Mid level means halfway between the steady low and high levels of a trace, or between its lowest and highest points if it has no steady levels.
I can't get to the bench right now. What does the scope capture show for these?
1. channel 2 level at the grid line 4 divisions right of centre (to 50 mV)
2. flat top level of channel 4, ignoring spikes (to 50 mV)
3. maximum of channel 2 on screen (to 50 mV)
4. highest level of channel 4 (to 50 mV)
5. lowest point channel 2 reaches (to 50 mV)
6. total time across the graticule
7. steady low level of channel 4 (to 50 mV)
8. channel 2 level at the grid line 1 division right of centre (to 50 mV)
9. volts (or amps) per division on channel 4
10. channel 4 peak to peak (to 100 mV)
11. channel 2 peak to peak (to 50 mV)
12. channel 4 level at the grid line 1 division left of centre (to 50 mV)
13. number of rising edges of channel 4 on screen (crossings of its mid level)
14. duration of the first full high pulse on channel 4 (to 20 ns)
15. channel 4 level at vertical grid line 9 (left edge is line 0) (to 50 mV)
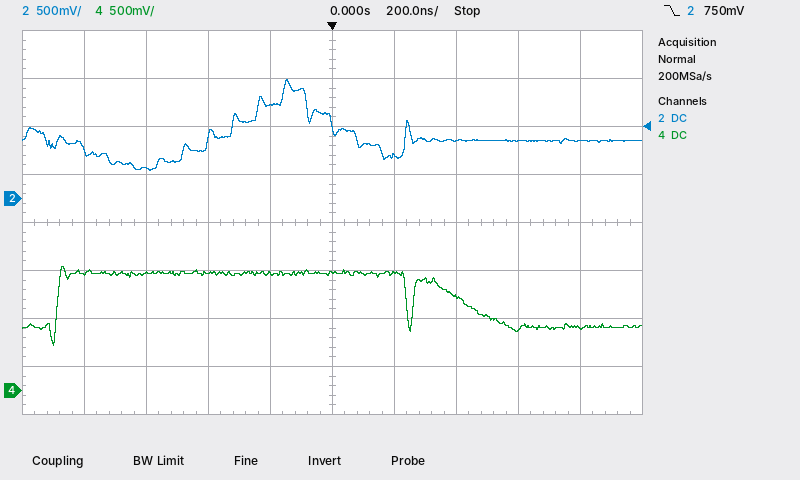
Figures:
600 mV
1.20 V
1.25 V
1.30 V
300 mV
2 µs
650 mV
450 mV
500 mV
800 mV
950 mV
1.20 V
2
1.12 µs
650 mV
